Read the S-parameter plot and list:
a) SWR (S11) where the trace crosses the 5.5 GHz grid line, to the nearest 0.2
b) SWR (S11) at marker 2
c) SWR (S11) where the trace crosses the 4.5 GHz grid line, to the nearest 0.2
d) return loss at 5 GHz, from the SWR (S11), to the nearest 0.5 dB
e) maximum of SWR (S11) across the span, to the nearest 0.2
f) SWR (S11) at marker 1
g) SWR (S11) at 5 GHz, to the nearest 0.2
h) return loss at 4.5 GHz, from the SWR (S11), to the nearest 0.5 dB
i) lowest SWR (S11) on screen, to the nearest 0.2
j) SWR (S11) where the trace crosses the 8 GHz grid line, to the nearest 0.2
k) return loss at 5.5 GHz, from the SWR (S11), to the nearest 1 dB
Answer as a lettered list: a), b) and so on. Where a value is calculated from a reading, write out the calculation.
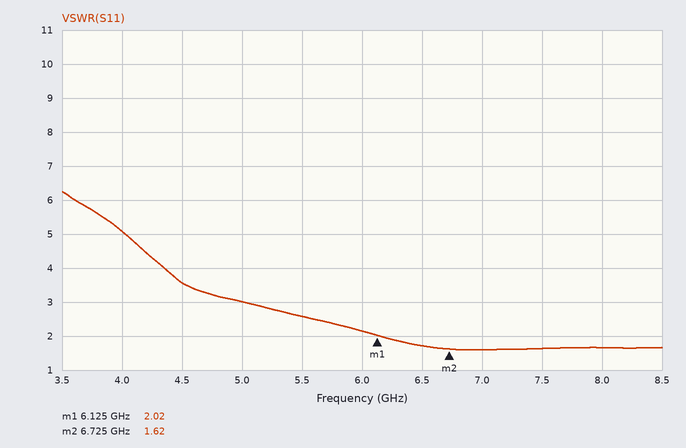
a) 2.6
b) 1.62
c) 3.6
d) −20 log10((3 − 1)/(3 + 1)) ≈ 6.0 dB
e) 6.2
f) 2.02
g) 3.0
h) −20 log10((3.6 − 1)/(3.6 + 1)) ≈ 5.0 dB
i) 1.6
j) 1.6
k) −20 log10((2.6 − 1)/(2.6 + 1)) ≈ 7 dB
